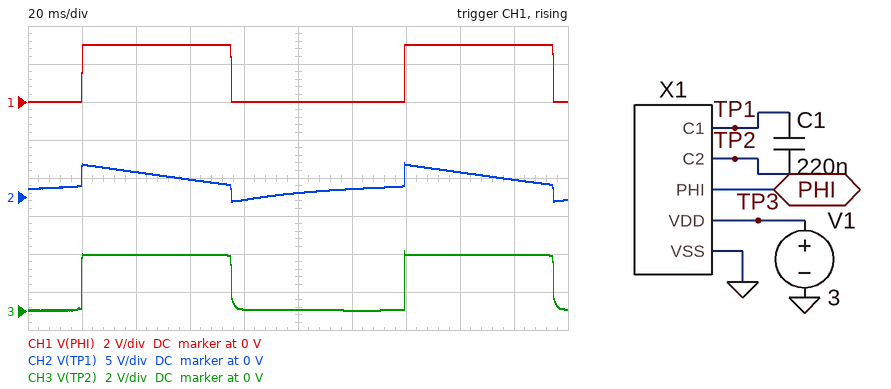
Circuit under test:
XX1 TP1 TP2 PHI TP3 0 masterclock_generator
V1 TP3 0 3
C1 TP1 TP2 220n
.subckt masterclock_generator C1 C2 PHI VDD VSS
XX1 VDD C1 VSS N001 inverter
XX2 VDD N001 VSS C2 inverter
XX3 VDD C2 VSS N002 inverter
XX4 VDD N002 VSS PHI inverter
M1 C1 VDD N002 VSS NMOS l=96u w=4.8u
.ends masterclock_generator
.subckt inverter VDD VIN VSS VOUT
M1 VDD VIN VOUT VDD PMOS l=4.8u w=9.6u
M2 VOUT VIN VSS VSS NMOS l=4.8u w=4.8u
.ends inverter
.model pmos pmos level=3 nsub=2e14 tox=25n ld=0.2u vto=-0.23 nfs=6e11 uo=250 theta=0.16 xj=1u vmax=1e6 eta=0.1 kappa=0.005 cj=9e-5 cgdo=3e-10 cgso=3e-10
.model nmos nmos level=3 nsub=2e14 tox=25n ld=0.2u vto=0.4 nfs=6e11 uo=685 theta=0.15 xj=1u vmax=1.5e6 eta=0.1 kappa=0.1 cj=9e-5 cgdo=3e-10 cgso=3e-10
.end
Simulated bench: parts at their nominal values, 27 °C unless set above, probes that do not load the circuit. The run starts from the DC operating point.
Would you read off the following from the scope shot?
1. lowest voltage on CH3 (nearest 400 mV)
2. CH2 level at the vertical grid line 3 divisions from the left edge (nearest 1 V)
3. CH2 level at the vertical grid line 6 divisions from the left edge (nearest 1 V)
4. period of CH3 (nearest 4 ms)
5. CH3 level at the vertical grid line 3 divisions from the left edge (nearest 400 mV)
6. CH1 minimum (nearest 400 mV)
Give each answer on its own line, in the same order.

0 V
2 V
1 V
120 ms
2.8 V
0 V
